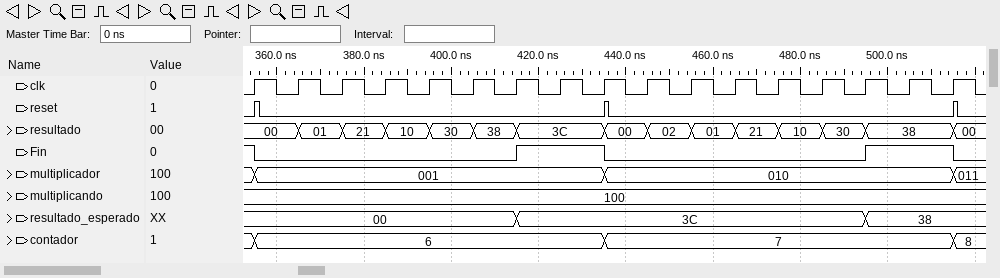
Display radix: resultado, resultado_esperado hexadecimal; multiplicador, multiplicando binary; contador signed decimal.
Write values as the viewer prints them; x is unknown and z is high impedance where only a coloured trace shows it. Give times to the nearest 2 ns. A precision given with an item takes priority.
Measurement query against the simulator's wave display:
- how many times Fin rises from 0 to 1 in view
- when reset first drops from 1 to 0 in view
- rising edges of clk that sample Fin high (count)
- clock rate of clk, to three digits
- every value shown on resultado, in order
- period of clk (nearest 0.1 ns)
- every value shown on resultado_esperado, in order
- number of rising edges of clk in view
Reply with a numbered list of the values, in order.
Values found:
1. 2
2. 356 ns
3. 5
4. 100 MHz
5. 00, 01, 21, 10, 30, 38, 3C, 00, 02, 01, 21, 10, 30, 38, 00
6. 10 ns
7. 00, 3C, 38
8. 17
